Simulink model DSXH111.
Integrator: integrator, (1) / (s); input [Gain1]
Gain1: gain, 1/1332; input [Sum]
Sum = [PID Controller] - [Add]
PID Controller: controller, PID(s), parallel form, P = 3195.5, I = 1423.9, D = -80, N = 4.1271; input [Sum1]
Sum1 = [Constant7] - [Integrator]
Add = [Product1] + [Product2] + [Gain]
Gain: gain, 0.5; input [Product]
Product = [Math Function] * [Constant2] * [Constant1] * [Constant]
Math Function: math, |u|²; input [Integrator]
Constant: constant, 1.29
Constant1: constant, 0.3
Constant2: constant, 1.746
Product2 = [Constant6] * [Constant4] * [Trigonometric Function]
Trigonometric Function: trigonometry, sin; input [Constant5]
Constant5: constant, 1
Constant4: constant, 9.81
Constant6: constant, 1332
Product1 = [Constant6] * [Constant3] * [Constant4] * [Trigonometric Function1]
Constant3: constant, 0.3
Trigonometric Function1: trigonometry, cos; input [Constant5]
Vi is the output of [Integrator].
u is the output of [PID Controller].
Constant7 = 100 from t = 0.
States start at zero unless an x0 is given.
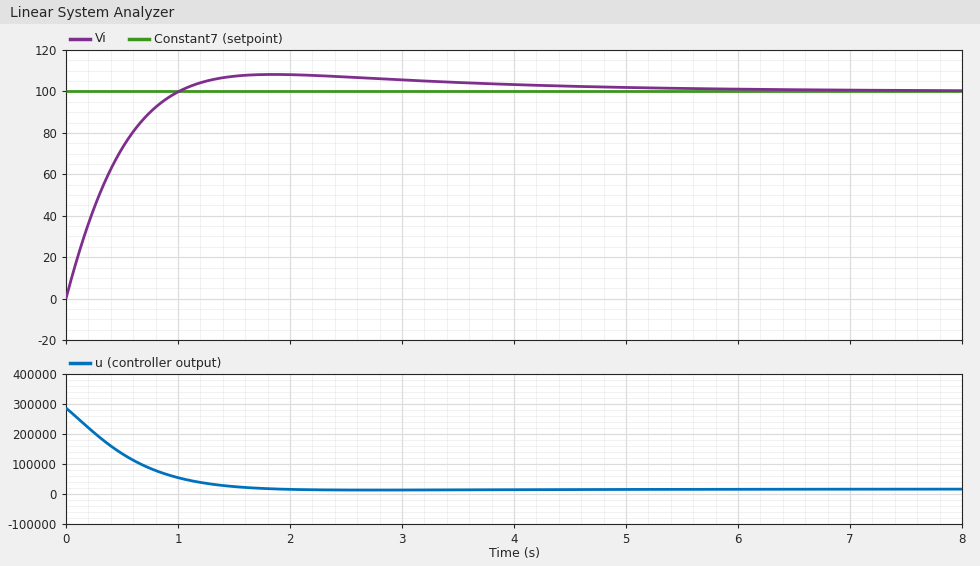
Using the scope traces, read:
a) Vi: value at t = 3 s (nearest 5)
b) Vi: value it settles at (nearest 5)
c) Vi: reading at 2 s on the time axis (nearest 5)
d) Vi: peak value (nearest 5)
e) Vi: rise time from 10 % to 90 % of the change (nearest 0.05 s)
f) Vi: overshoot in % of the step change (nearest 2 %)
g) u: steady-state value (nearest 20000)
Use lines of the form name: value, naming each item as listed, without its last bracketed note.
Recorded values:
Vi: value at t = 3 s: 105
Vi: value it settles at: 100
Vi: reading at 2 s on the time axis: 110
Vi: peak value: 110
Vi: rise time from 10 % to 90 % of the change: 0.70 s
Vi: overshoot in % of the step change: 8 %
u: steady-state value: 20000
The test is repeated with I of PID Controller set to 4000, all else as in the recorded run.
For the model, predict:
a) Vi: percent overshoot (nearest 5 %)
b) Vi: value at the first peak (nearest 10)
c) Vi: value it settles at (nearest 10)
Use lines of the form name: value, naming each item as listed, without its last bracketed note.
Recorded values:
Vi: percent overshoot: 20 %
Vi: value at the first peak: 120
Vi: value it settles at: 100
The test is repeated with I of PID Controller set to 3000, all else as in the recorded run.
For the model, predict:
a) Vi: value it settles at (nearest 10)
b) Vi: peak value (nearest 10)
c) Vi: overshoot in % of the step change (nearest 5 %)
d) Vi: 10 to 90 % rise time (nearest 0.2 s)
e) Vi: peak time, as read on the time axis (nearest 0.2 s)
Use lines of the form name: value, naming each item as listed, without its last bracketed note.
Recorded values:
Vi: value it settles at: 100
Vi: peak value: 120
Vi: overshoot in % of the step change: 15 %
Vi: 10 to 90 % rise time: 0.6 s
Vi: peak time, as read on the time axis: 1.4 s
